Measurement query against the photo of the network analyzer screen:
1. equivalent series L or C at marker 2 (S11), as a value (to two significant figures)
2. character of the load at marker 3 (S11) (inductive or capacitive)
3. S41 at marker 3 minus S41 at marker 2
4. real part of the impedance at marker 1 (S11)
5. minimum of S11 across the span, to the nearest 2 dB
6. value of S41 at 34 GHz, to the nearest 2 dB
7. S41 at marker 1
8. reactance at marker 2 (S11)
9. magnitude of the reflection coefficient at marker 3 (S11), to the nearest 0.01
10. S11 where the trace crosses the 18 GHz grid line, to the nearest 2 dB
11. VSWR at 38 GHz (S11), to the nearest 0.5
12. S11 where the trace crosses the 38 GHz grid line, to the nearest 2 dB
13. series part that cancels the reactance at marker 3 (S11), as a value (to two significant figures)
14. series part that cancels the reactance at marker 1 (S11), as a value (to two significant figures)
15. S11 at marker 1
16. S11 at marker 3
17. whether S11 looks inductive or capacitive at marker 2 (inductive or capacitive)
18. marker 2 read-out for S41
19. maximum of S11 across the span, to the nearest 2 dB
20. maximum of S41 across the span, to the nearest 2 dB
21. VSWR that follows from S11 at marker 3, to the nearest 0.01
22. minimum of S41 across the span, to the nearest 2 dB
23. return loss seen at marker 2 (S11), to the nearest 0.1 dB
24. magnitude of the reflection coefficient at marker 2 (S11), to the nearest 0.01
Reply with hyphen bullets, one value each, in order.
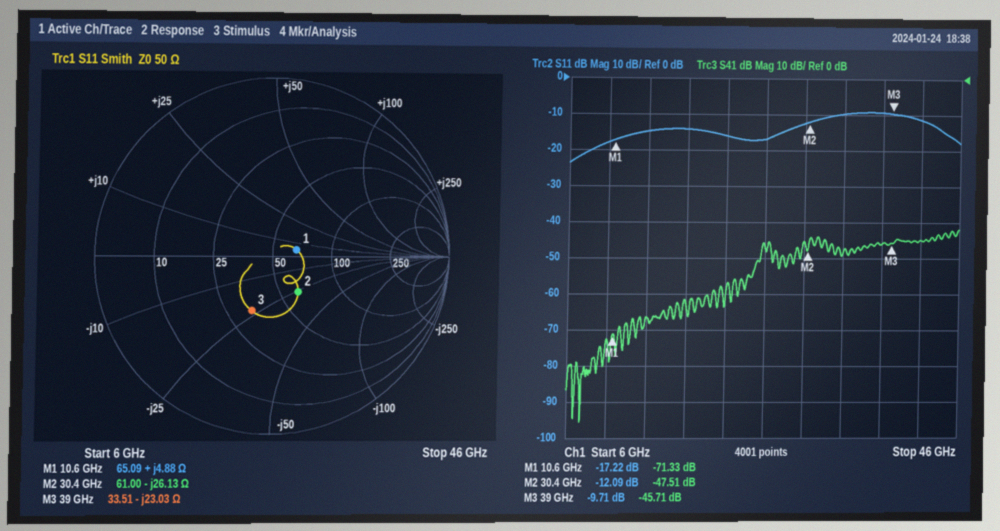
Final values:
- 200 fF
- capacitive
- 1.80 dB
- 65.09 Ω
- -24 dB
- -48 dB
- -71.33 dB
- -26.13 Ω
- 0.33
- -14 dB
- 2.0
- -10 dB
- 94 pH
- 3.1 pF
- -17.22 dB
- -9.71 dB
- capacitive
- -47.51 dB
- -10 dB
- -42 dB
- 1.97
- -96 dB
- 12.1 dB
- 0.25
